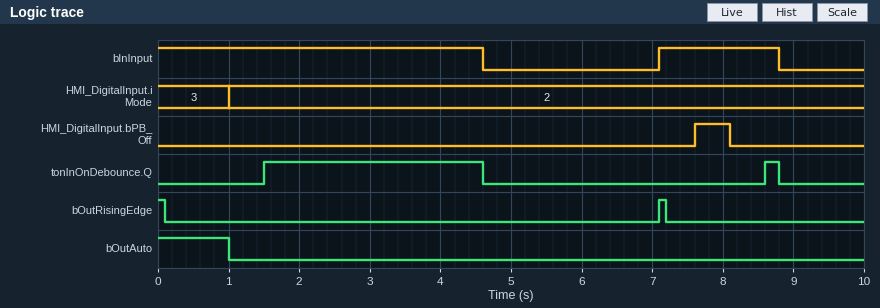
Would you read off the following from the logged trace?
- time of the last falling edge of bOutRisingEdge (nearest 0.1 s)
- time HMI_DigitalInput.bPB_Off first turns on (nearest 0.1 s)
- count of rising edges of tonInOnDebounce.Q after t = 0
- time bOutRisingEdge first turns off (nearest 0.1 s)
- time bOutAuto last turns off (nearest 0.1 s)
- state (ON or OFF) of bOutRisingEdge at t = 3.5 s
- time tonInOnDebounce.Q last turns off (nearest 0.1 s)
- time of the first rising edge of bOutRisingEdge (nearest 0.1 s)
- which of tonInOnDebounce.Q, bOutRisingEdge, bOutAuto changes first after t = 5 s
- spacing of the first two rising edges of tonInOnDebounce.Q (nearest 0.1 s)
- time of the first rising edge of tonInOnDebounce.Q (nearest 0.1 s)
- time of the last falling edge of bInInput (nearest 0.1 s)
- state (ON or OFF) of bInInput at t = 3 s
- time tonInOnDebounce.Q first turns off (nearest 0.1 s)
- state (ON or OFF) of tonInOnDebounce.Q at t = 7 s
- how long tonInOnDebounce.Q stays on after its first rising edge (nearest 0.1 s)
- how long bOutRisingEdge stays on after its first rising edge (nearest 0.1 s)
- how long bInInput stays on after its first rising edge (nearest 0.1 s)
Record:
7.2 s
7.6 s
2
0.1 s
1.0 s
OFF
8.8 s
7.1 s
bOutRisingEdge
7.1 s
1.5 s
8.8 s
ON
4.6 s
OFF
3.1 s
0.1 s
1.7 s
